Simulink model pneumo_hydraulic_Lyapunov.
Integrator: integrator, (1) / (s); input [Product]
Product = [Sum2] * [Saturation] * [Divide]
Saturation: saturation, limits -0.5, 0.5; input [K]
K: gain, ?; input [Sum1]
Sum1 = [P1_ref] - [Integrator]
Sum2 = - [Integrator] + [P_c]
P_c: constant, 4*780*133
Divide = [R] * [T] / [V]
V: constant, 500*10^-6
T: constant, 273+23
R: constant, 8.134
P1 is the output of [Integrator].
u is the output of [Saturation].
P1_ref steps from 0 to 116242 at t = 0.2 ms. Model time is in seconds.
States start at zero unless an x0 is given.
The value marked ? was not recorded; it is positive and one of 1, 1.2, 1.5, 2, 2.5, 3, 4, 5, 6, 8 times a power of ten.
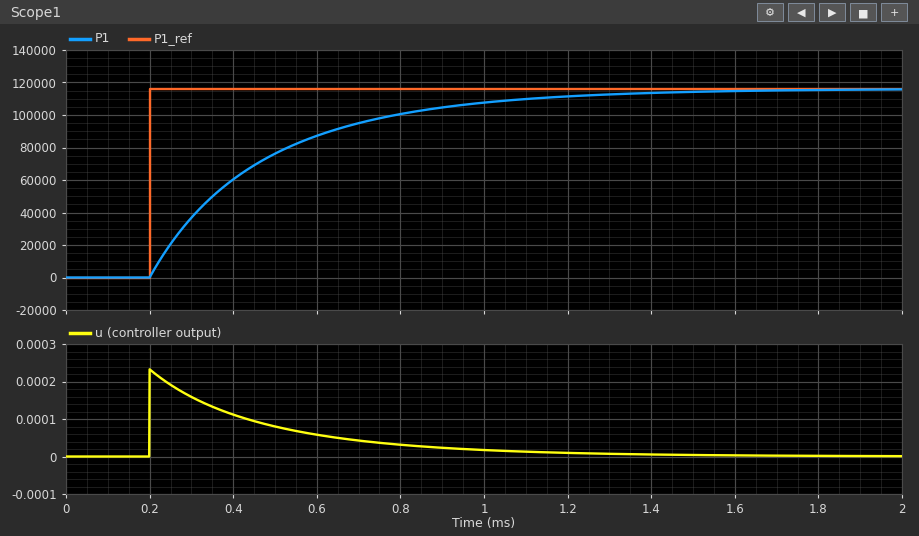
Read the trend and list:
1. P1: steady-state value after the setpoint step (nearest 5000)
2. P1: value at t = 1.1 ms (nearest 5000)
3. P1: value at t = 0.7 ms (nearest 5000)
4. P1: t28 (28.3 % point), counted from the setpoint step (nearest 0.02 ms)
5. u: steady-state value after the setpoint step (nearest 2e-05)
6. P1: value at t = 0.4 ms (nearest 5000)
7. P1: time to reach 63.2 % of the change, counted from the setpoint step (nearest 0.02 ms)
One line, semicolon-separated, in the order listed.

115000; 110000; 95000; 0.08 ms; 0.00000; 60000; 0.28 ms
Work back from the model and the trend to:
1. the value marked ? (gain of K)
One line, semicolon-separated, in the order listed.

2e-09
